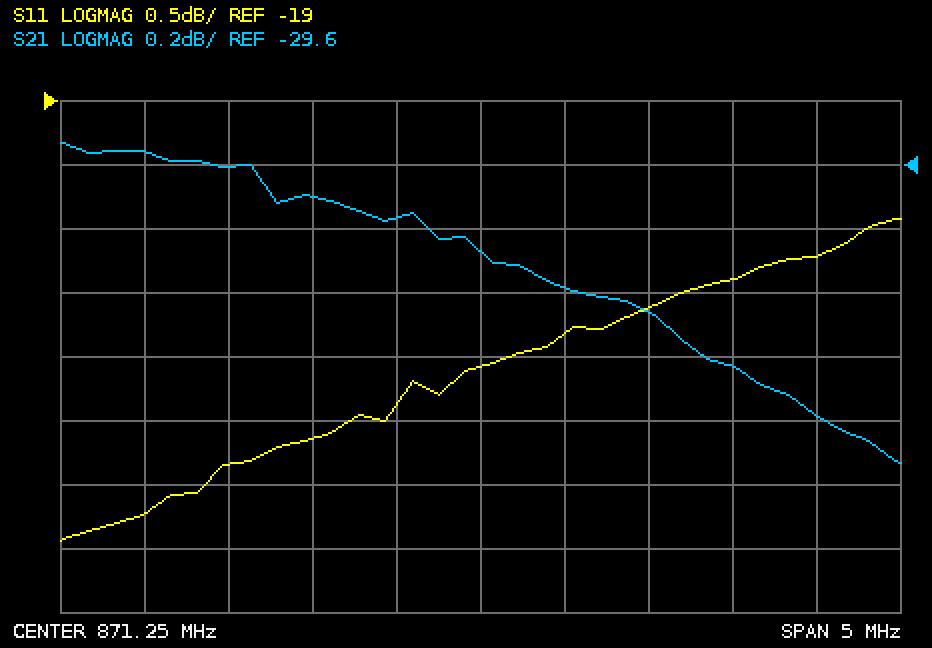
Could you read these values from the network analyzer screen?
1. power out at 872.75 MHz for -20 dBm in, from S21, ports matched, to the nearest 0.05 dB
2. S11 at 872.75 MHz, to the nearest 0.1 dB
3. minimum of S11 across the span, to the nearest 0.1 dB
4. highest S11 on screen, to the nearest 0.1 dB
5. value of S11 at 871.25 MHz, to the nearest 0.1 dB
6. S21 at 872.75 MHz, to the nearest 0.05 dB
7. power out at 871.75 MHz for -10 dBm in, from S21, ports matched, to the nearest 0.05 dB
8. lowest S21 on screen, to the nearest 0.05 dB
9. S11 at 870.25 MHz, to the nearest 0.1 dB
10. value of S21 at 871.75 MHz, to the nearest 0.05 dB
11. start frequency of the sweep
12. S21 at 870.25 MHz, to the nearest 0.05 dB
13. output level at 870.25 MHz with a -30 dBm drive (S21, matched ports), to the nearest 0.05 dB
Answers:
-50.25 dBm
-20.4 dB
-22.4 dB
-19.9 dB
-21.1 dB
-30.25 dB
-40.00 dBm
-30.55 dB
-21.6 dB
-30.00 dB
868.75 MHz
-29.70 dB
-59.70 dBm
